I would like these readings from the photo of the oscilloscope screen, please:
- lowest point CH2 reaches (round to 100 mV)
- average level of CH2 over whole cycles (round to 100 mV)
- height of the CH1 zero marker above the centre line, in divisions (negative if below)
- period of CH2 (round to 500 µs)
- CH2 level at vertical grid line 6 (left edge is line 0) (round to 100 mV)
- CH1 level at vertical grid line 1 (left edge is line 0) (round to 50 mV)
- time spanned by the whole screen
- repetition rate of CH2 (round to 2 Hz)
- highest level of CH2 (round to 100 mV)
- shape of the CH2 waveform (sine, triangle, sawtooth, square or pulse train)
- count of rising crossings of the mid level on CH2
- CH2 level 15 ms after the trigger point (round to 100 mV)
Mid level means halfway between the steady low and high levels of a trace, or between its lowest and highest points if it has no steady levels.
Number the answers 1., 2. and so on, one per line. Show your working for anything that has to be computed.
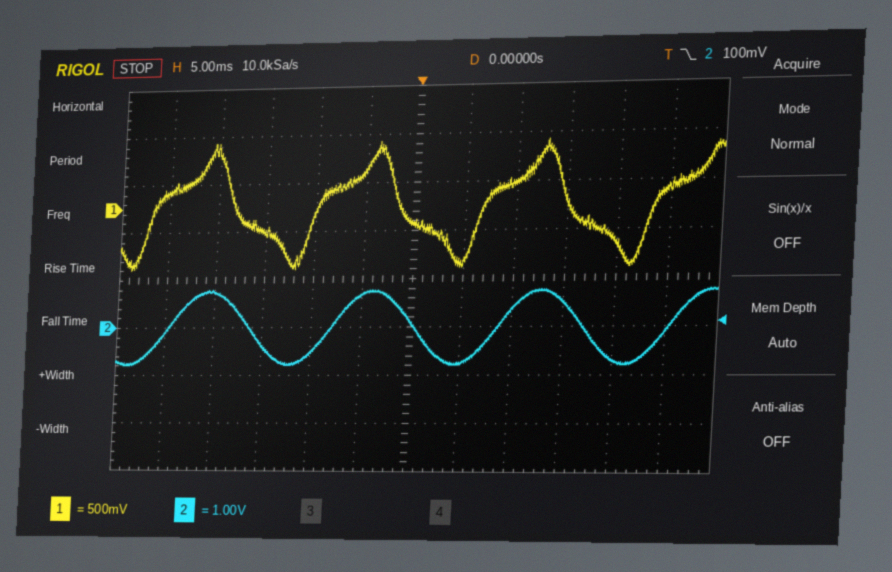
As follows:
1. -800 mV
2. (800 mV + (-800 mV)) / 2 ≈ 0.0 V
3. +1.5 div
4. 16.5 ms
5. 100 mV
6. 150 mV
7. 60 ms
8. 1 / 16.5 ms ≈ 60.6 Hz, so 60 Hz to the nearest 2 Hz
9. 800 mV
10. sine
11. 4
12. 500 mV
